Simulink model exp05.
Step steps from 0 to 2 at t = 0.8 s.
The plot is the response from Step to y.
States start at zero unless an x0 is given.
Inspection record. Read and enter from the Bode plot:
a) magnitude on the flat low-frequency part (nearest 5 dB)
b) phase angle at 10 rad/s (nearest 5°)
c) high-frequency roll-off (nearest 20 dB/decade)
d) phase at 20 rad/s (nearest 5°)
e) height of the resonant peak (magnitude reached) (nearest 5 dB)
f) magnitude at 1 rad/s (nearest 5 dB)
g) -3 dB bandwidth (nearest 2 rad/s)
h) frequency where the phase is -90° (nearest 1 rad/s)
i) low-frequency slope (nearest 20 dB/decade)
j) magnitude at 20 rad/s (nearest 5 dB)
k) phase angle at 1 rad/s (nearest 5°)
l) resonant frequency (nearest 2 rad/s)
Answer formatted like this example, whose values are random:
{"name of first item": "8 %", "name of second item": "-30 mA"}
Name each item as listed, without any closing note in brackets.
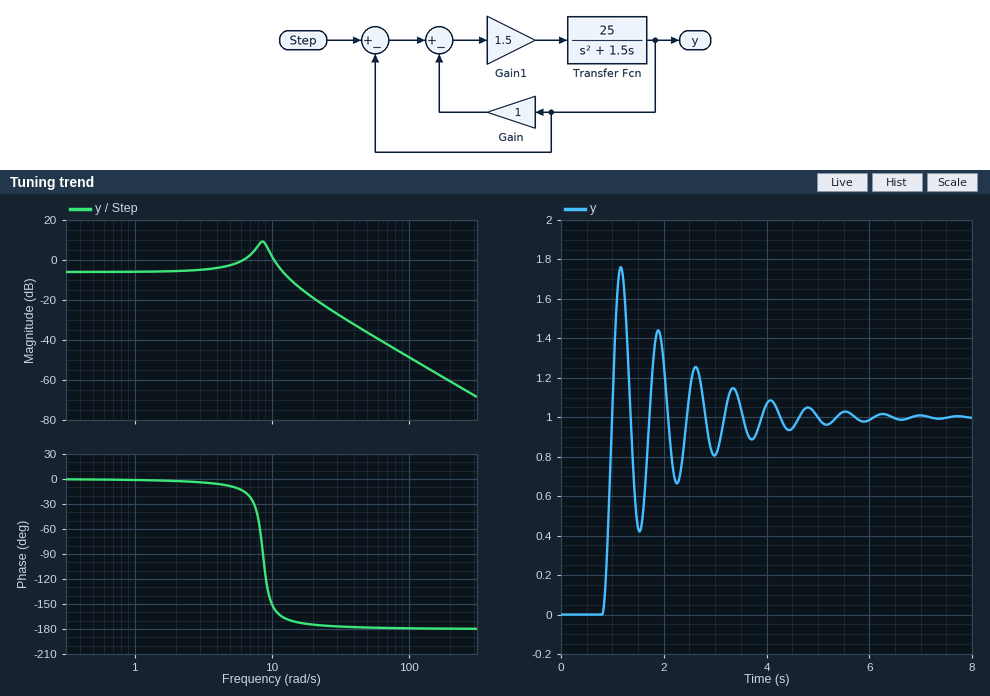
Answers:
{"magnitude on the flat low-frequency part": "-5 dB", "phase angle at 10 rad/s": "-150°", "high-frequency roll-off": "-40 dB/decade", "phase at 20 rad/s": "-175°", "height of the resonant peak (magnitude reached)": "10 dB", "magnitude at 1 rad/s": "-5 dB", "-3 dB bandwidth": "14 rad/s", "frequency where the phase is -90°": "9 rad/s", "low-frequency slope": "0 dB/decade", "magnitude at 20 rad/s": "-20 dB", "phase angle at 1 rad/s": "0°", "resonant frequency": "8 rad/s"}
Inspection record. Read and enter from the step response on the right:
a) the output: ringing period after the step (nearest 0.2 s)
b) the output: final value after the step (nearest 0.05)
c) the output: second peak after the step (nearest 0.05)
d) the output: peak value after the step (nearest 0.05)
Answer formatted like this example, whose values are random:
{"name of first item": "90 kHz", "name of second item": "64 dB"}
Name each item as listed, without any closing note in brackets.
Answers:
{"the output: ringing period after the step": "0.8 s", "the output: final value after the step": "1.00", "the output: second peak after the step": "1.45", "the output: peak value after the step": "1.75"}
